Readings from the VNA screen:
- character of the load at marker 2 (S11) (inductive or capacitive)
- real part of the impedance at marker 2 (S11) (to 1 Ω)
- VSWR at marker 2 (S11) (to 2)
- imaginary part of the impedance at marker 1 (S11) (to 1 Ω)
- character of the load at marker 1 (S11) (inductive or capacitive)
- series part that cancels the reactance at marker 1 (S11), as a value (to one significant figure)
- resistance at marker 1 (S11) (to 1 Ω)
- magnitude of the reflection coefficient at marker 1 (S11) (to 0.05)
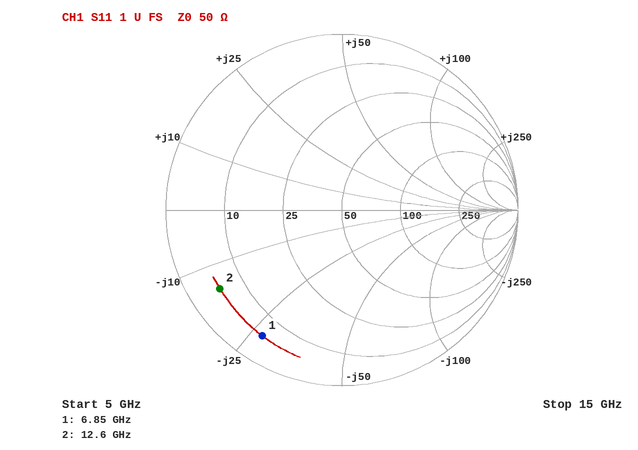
capacitive
5 Ω
10
-27 Ω
capacitive
600 pH
5 Ω
0.85
